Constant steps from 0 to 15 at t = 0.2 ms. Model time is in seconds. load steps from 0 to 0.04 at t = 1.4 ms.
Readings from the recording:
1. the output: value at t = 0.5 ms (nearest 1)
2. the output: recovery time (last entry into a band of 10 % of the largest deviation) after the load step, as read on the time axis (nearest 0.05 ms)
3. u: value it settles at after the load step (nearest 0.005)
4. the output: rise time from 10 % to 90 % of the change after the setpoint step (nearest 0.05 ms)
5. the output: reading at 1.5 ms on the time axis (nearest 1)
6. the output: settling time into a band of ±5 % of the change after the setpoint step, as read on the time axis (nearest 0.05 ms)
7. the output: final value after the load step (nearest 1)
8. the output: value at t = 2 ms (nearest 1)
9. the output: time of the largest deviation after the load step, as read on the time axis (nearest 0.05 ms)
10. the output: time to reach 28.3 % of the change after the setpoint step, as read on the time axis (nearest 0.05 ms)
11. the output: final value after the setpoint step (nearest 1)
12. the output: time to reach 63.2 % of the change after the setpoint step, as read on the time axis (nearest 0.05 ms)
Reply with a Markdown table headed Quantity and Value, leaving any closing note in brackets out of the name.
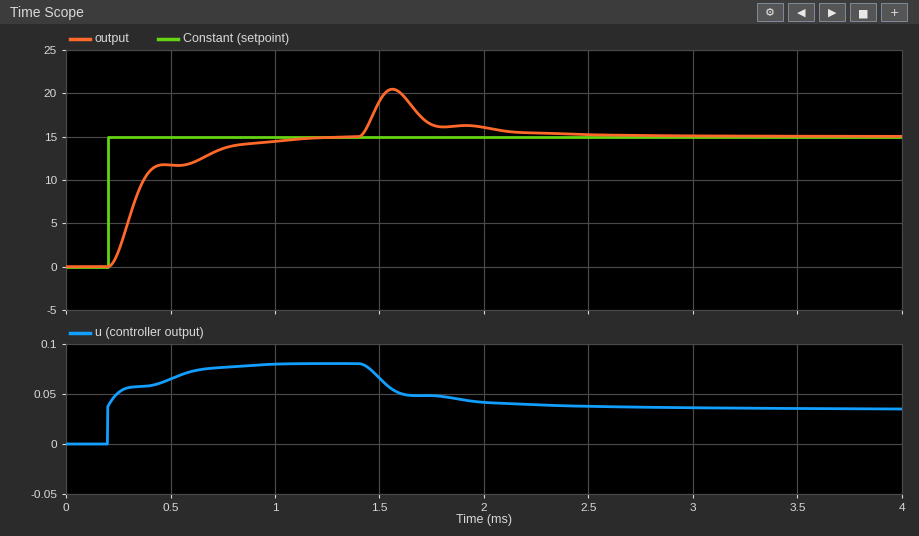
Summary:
| Quantity | Value |
|---|---|
| the output: value at t = 0.5 ms | 12 |
| the output: recovery time (last entry into a band of 10 % of the largest deviation) after the load step, as read on the time axis | 2.15 ms |
| u: value it settles at after the load step | 0.035 |
| the output: rise time from 10 % to 90 % of the change after the setpoint step | 0.50 ms |
| the output: reading at 1.5 ms on the time axis | 19 |
| the output: settling time into a band of ±5 % of the change after the setpoint step, as read on the time axis | 0.90 ms |
| the output: final value after the load step | 15 |
| the output: value at t = 2 ms | 16 |
| the output: time of the largest deviation after the load step, as read on the time axis | 1.55 ms |
| the output: time to reach 28.3 % of the change after the setpoint step, as read on the time axis | 0.30 ms |
| the output: final value after the setpoint step | 15 |
| the output: time to reach 63.2 % of the change after the setpoint step, as read on the time axis | 0.35 ms |
